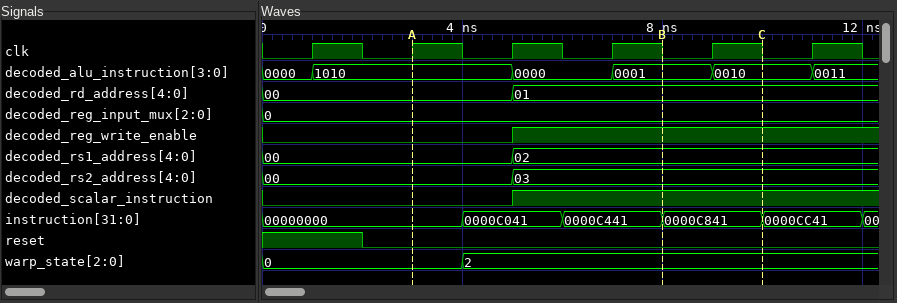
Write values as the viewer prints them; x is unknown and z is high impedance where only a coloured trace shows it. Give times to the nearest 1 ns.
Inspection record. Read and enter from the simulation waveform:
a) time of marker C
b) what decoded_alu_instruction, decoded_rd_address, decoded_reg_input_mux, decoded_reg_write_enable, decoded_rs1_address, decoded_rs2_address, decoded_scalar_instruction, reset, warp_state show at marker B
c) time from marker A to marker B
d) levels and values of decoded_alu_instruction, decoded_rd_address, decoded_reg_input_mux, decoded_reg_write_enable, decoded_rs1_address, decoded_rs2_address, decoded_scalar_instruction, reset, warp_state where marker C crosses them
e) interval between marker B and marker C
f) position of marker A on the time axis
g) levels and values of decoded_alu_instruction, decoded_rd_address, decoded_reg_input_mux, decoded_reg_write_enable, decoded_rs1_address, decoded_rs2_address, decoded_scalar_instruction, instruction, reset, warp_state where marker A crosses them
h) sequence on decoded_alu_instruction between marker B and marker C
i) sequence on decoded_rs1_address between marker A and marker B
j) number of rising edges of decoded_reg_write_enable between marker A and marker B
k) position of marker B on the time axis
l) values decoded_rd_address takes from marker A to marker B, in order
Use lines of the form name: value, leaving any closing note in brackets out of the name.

time of marker C: 10 ns
what decoded_alu_instruction, decoded_rd_address, decoded_reg_input_mux, decoded_reg_write_enable, decoded_rs1_address, decoded_rs2_address, decoded_scalar_instruction, reset, warp_state show at marker B: decoded_alu_instruction=0001, decoded_rd_address=01, decoded_reg_input_mux=0, decoded_reg_write_enable=1, decoded_rs1_address=02, decoded_rs2_address=03, decoded_scalar_instruction=1, reset=0, warp_state=2
time from marker A to marker B: 5 ns
levels and values of decoded_alu_instruction, decoded_rd_address, decoded_reg_input_mux, decoded_reg_write_enable, decoded_rs1_address, decoded_rs2_address, decoded_scalar_instruction, reset, warp_state where marker C crosses them: decoded_alu_instruction=0010, decoded_rd_address=01, decoded_reg_input_mux=0, decoded_reg_write_enable=1, decoded_rs1_address=02, decoded_rs2_address=03, decoded_scalar_instruction=1, reset=0, warp_state=2
interval between marker B and marker C: 2 ns
position of marker A on the time axis: 3 ns
levels and values of decoded_alu_instruction, decoded_rd_address, decoded_reg_input_mux, decoded_reg_write_enable, decoded_rs1_address, decoded_rs2_address, decoded_scalar_instruction, instruction, reset, warp_state where marker A crosses them: decoded_alu_instruction=1010, decoded_rd_address=00, decoded_reg_input_mux=0, decoded_reg_write_enable=0, decoded_rs1_address=00, decoded_rs2_address=00, decoded_scalar_instruction=0, instruction=00000000, reset=0, warp_state=0
sequence on decoded_alu_instruction between marker B and marker C: 0001, 0010
sequence on decoded_rs1_address between marker A and marker B: 00, 02
number of rising edges of decoded_reg_write_enable between marker A and marker B: 1
position of marker B on the time axis: 8 ns
values decoded_rd_address takes from marker A to marker B, in order: 00, 01
